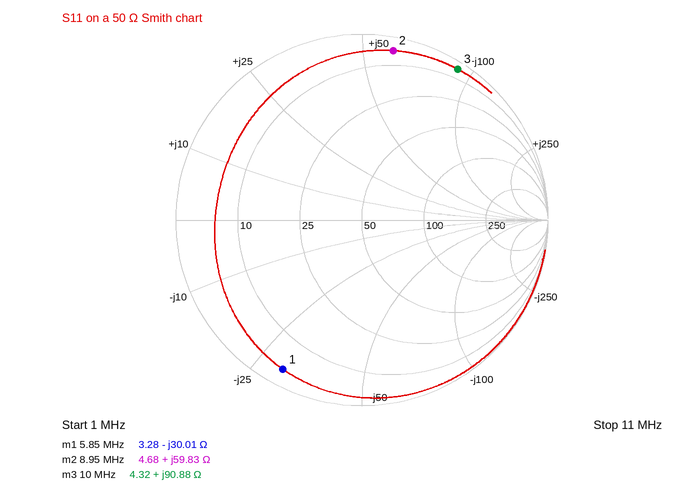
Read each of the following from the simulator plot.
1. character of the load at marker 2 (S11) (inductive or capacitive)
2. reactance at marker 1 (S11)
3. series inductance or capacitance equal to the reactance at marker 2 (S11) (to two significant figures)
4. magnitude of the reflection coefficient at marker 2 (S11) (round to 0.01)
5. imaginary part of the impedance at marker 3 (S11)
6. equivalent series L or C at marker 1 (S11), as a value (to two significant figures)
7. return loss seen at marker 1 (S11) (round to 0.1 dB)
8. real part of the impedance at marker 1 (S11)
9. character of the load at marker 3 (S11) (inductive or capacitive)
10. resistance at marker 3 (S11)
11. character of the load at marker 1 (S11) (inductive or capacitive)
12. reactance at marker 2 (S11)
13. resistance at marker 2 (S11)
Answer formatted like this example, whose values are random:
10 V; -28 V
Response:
inductive; -30.01 Ω; 1.1 µH; 0.93; +90.88 Ω; 910 pF; 0.8 dB; 3.28 Ω; inductive; 4.32 Ω; capacitive; +59.83 Ω; 4.68 Ω
